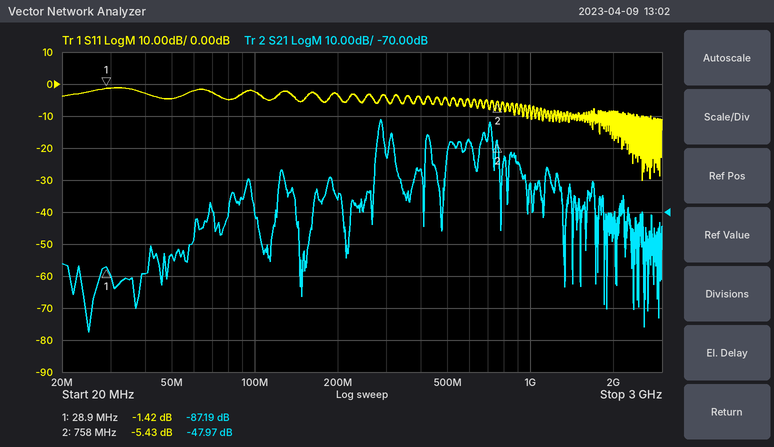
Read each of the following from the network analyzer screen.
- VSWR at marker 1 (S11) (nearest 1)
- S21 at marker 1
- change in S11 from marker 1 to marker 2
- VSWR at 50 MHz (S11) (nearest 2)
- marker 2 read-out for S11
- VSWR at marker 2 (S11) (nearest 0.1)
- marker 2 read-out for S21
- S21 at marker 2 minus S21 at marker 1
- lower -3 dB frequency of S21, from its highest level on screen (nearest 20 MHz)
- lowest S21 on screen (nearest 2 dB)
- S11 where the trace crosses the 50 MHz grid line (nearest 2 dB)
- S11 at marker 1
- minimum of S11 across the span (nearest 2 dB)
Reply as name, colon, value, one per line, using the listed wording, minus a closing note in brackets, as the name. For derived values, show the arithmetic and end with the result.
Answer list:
VSWR at marker 1 (S11): (1 + 0.8492)/(1 − 0.8492) ≈ 12
S21 at marker 1: -87.19 dB
change in S11 from marker 1 to marker 2: -5.43 − (-1.42) = -4.01 dB
VSWR at 50 MHz (S11): |Γ| = 10^(-4/20) = 0.6310; VSWR = (1 + 0.6310)/(1 − 0.6310) ≈ 4
marker 2 read-out for S11: -5.43 dB
VSWR at marker 2 (S11): (1 + 0.5352)/(1 − 0.5352) ≈ 3.3
marker 2 read-out for S21: -47.97 dB
S21 at marker 2 minus S21 at marker 1: -47.97 − (-87.19) = 39.22 dB
lower -3 dB frequency of S21, from its highest level on screen: 280 MHz
lowest S21 on screen: -108 dB
S11 where the trace crosses the 50 MHz grid line: -4 dB
S11 at marker 1: -1.42 dB
minimum of S11 across the span: -30 dB
